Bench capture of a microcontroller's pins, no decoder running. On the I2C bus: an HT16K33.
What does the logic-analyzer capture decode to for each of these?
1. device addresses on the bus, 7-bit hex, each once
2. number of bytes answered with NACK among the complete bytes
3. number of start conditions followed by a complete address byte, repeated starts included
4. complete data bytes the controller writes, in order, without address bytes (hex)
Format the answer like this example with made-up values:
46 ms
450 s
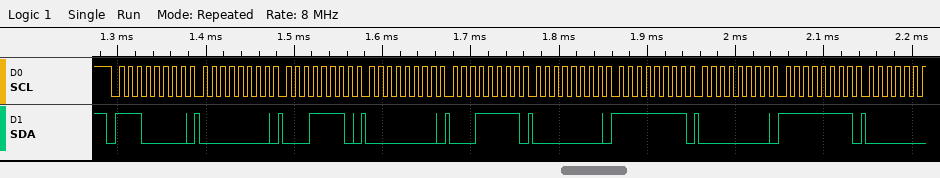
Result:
0x70
0
1
00 1E 00 1F 00 FF 00 FF
